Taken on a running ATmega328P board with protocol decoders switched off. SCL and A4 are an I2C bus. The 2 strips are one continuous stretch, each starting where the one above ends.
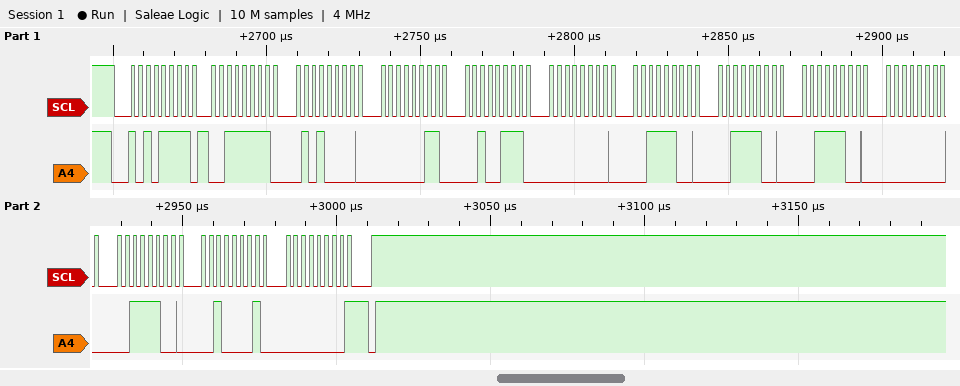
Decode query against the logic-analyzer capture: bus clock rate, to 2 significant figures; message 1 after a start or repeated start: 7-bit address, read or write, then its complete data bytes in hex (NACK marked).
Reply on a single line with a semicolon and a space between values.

400 kHz; 0x57 read: 3F 50 03 27 00 3C 3C 3C 00 3C 21 00 NACK
